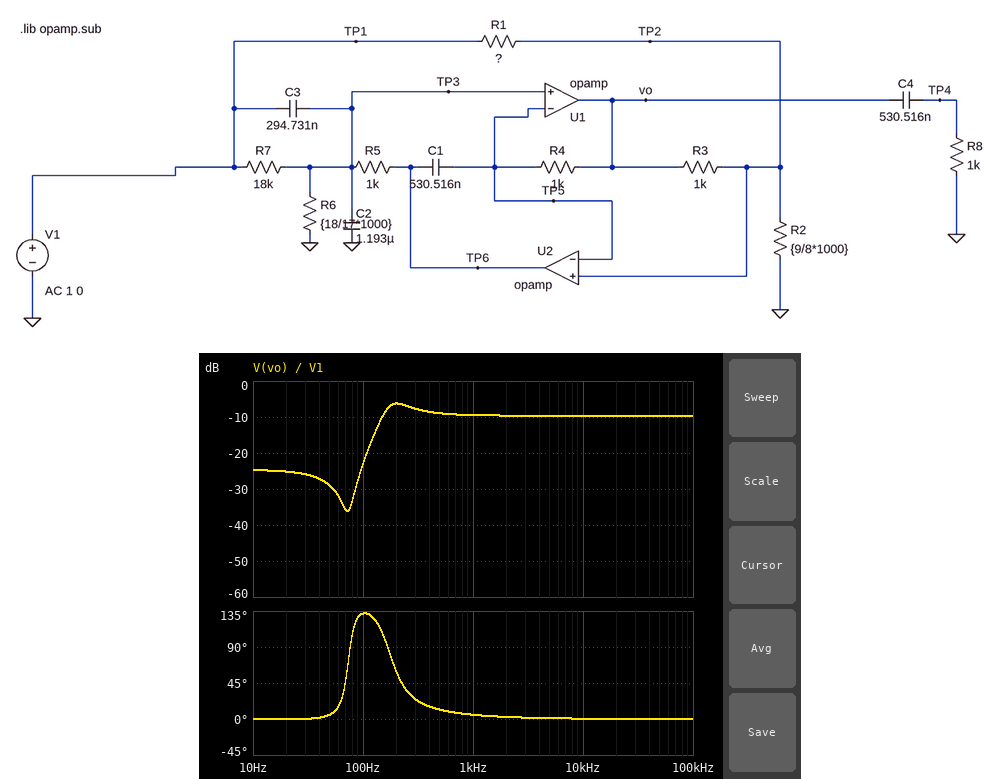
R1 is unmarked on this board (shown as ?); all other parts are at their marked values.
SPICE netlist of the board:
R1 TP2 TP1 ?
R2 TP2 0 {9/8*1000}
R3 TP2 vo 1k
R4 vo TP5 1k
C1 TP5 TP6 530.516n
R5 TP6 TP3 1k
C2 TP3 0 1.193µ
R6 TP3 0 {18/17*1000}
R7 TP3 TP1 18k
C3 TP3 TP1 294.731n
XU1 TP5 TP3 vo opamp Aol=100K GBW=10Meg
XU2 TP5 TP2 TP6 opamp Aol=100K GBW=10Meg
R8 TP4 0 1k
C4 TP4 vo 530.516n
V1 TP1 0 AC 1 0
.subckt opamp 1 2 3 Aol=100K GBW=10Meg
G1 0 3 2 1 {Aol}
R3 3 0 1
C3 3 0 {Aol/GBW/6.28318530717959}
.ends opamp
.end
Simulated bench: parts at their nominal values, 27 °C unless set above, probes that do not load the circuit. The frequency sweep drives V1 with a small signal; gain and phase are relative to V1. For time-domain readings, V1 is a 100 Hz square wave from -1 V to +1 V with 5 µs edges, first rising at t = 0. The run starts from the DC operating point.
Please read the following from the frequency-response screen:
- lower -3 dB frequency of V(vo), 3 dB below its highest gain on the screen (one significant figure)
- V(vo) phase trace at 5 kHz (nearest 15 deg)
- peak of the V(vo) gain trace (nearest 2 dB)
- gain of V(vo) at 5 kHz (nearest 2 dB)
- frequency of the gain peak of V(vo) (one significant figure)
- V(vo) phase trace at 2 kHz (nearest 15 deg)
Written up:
200 Hz
0 deg
-6 dB
-10 dB
200 Hz
0 deg
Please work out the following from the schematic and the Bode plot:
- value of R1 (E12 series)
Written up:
18 kΩ
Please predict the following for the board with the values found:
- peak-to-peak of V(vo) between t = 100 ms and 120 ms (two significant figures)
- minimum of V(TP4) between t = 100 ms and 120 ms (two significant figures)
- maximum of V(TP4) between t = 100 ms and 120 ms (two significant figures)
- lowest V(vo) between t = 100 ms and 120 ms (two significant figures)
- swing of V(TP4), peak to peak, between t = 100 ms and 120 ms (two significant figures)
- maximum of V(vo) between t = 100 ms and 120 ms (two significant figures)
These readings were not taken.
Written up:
1.0 V
-610 mV
610 mV
-520 mV
1.2 V
520 mV
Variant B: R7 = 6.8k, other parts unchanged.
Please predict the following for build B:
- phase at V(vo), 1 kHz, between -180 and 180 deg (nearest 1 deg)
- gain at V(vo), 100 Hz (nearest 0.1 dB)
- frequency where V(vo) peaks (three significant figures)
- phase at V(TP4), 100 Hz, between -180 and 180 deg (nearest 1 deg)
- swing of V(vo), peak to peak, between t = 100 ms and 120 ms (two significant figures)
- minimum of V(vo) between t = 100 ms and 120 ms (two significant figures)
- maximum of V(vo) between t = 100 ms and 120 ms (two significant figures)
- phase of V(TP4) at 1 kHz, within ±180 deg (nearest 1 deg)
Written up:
3 deg
-18.3 dB
202 Hz
164 deg
1.1 V
-560 mV
560 mV
19 deg
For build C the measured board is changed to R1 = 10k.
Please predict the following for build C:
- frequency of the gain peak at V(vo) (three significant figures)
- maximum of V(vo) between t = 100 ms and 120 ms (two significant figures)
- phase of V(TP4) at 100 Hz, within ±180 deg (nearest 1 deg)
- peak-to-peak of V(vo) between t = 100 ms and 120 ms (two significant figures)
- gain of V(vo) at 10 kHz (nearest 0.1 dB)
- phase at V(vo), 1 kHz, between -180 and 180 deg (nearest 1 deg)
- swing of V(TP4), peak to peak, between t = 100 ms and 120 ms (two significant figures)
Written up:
219 Hz
410 mV
68 deg
830 mV
-10.6 dB
6 deg
1.1 V
